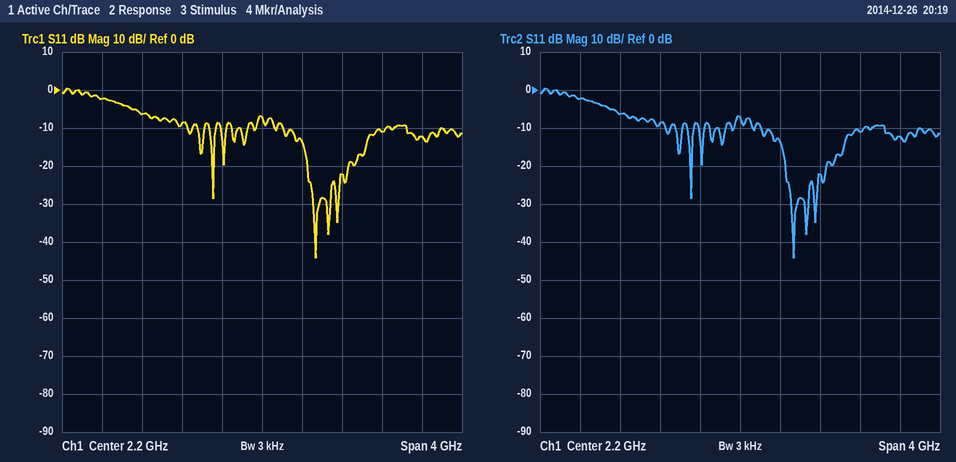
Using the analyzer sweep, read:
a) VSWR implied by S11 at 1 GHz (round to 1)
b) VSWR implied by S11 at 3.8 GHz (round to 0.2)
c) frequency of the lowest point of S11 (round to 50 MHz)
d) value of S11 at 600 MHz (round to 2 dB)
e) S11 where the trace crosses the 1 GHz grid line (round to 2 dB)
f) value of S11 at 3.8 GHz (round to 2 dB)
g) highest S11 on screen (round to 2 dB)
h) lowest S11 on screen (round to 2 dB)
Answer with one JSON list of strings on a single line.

["3", "1.6", "2.75 GHz", "-2 dB", "-6 dB", "-12 dB", "0 dB", "-44 dB"]
